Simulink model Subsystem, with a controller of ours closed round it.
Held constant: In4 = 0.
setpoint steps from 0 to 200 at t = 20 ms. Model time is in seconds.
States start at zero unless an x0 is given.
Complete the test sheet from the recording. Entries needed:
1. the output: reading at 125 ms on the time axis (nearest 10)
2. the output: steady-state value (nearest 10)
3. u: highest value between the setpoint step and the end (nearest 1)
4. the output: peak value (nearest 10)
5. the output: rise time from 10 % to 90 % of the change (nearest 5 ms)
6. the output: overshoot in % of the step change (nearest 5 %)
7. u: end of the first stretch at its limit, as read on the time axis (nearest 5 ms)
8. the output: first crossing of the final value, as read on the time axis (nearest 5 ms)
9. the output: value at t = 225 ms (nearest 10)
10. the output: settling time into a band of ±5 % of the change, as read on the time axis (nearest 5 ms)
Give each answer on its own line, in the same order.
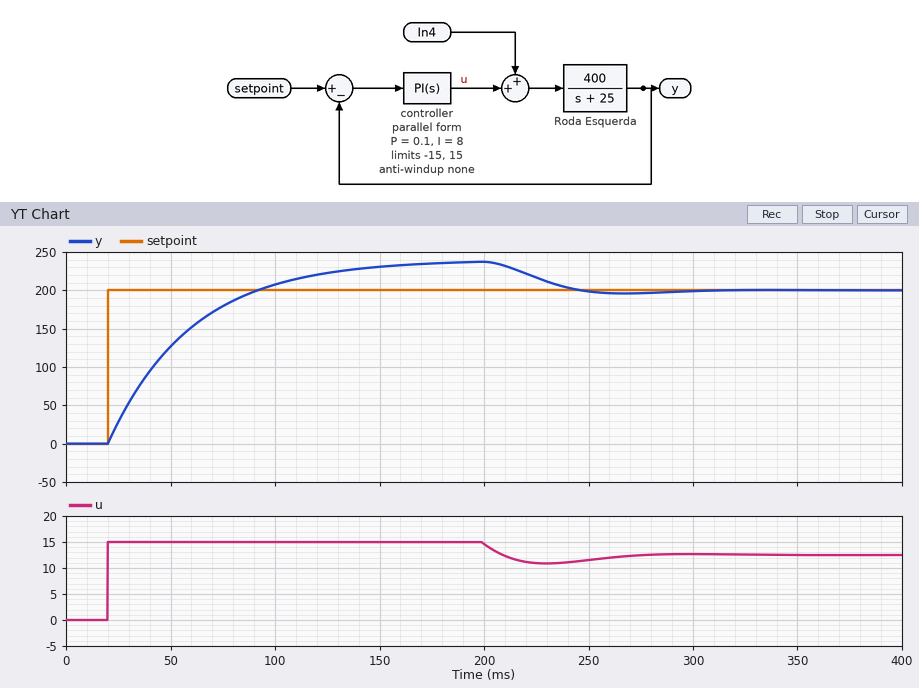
220
200
15
240
50 ms
20 %
200 ms
90 ms
220
230 ms
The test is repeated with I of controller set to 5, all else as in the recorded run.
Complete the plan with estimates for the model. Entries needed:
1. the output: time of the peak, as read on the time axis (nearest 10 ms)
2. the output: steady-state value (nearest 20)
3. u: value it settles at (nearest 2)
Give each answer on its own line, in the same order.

160 ms
200
12
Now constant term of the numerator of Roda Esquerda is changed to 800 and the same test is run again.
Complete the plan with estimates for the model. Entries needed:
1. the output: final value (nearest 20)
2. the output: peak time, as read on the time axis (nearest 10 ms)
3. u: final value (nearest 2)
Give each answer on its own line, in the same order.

200
60 ms
6
